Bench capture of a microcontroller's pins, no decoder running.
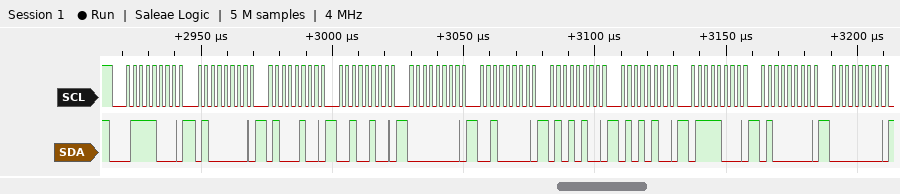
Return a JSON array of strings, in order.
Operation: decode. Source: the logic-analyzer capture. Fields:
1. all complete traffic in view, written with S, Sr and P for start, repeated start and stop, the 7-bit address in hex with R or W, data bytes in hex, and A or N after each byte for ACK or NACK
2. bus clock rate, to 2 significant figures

["S 3CW A 40 A 44 A 24 A 00 A 20 A 54 A 54 A 78 A 40 A 00 A", "400 kHz"]
